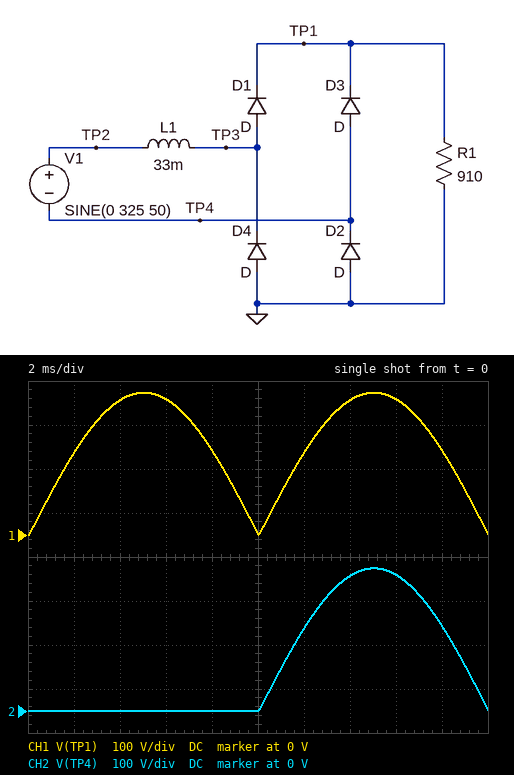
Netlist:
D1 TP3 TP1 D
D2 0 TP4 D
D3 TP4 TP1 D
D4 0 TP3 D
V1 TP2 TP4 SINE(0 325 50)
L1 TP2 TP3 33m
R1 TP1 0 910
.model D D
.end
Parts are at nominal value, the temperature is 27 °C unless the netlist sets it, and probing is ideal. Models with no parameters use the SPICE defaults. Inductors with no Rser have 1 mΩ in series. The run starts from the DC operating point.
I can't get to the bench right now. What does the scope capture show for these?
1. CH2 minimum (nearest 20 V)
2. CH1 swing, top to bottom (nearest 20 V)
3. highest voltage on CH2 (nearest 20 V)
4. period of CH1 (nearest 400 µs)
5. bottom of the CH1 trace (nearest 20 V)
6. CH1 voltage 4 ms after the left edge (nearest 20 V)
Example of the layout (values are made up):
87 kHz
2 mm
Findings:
0 V
320 V
320 V
10.0 ms
0 V
300 V
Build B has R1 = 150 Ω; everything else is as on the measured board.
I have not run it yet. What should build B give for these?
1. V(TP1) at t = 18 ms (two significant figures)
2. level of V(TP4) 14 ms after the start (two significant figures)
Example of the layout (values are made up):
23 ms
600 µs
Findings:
210 V
300 V
